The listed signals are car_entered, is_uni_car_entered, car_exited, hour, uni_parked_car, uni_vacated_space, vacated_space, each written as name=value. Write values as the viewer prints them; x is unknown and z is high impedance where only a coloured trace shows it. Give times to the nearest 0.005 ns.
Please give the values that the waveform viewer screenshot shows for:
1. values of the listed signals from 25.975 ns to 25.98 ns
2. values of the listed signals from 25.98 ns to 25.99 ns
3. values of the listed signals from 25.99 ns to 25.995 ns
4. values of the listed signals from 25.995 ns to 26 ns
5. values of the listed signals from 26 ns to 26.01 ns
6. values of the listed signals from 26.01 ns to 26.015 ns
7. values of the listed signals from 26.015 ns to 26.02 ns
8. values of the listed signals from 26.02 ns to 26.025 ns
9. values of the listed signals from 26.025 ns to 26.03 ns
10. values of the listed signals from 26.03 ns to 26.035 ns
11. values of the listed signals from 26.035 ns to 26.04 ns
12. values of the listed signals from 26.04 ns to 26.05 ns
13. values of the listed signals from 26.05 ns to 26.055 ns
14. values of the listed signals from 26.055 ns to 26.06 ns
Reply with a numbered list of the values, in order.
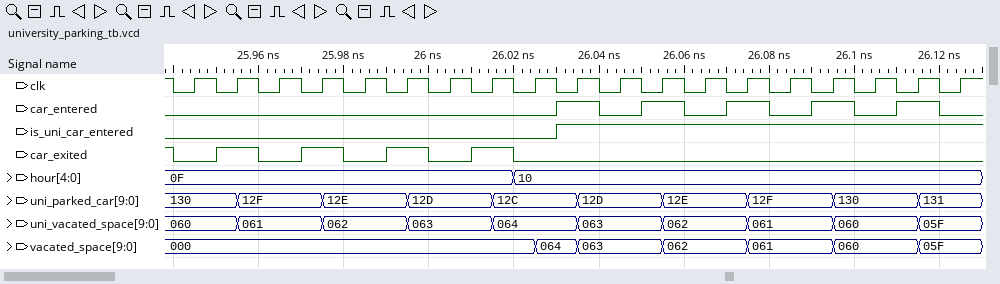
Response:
1. car_entered=0, is_uni_car_entered=0, car_exited=1, hour=0F, uni_parked_car=12E, uni_vacated_space=062, vacated_space=000
2. car_entered=0, is_uni_car_entered=0, car_exited=0, hour=0F, uni_parked_car=12E, uni_vacated_space=062, vacated_space=000
3. car_entered=0, is_uni_car_entered=0, car_exited=1, hour=0F, uni_parked_car=12E, uni_vacated_space=062, vacated_space=000
4. car_entered=0, is_uni_car_entered=0, car_exited=1, hour=0F, uni_parked_car=12D, uni_vacated_space=063, vacated_space=000
5. car_entered=0, is_uni_car_entered=0, car_exited=0, hour=0F, uni_parked_car=12D, uni_vacated_space=063, vacated_space=000
6. car_entered=0, is_uni_car_entered=0, car_exited=1, hour=0F, uni_parked_car=12D, uni_vacated_space=063, vacated_space=000
7. car_entered=0, is_uni_car_entered=0, car_exited=1, hour=0F, uni_parked_car=12C, uni_vacated_space=064, vacated_space=000
8. car_entered=0, is_uni_car_entered=0, car_exited=0, hour=10, uni_parked_car=12C, uni_vacated_space=064, vacated_space=000
9. car_entered=0, is_uni_car_entered=0, car_exited=0, hour=10, uni_parked_car=12C, uni_vacated_space=064, vacated_space=064
10. car_entered=1, is_uni_car_entered=1, car_exited=0, hour=10, uni_parked_car=12C, uni_vacated_space=064, vacated_space=064
11. car_entered=1, is_uni_car_entered=1, car_exited=0, hour=10, uni_parked_car=12D, uni_vacated_space=063, vacated_space=063
12. car_entered=0, is_uni_car_entered=1, car_exited=0, hour=10, uni_parked_car=12D, uni_vacated_space=063, vacated_space=063
13. car_entered=1, is_uni_car_entered=1, car_exited=0, hour=10, uni_parked_car=12D, uni_vacated_space=063, vacated_space=063
14. car_entered=1, is_uni_car_entered=1, car_exited=0, hour=10, uni_parked_car=12E, uni_vacated_space=062, vacated_space=062
